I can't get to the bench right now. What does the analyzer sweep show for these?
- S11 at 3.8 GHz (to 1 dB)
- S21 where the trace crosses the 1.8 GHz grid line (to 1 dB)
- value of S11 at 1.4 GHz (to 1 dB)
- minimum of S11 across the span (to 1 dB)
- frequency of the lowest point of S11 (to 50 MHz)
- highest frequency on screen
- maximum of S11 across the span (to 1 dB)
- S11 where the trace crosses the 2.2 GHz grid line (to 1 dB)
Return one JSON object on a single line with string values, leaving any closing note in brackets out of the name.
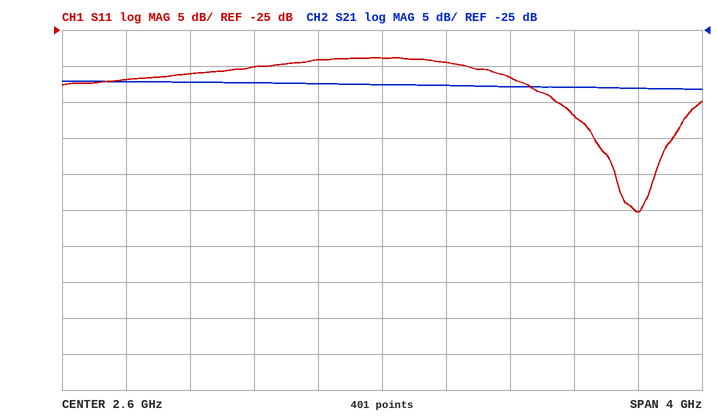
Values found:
{"S11 at 3.8 GHz": "-37 dB", "S21 where the trace crosses the 1.8 GHz grid line": "-32 dB", "value of S11 at 1.4 GHz": "-31 dB", "minimum of S11 across the span": "-50 dB", "frequency of the lowest point of S11": "4.20 GHz", "highest frequency on screen": "4.6 GHz", "maximum of S11 across the span": "-29 dB", "S11 where the trace crosses the 2.2 GHz grid line": "-29 dB"}
